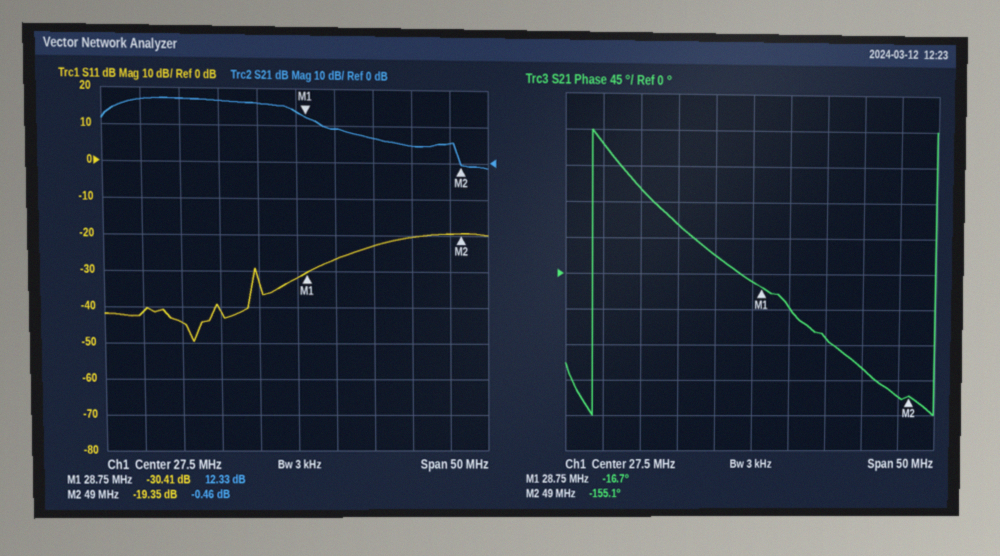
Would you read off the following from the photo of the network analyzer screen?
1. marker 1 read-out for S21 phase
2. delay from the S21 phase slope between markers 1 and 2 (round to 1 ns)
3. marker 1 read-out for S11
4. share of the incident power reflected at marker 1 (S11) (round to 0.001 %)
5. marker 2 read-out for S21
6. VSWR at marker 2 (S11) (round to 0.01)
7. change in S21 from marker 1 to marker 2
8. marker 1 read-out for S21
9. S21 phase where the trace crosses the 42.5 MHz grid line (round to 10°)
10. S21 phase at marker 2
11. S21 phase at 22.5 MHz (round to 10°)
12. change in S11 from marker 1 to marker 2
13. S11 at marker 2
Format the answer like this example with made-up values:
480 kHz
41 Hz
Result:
-16.7°
19 ns
-30.41 dB
0.091 %
-0.46 dB
1.24
-12.79 dB
12.33 dB
-120°
-155.1°
20°
11.06 dB
-19.35 dB
